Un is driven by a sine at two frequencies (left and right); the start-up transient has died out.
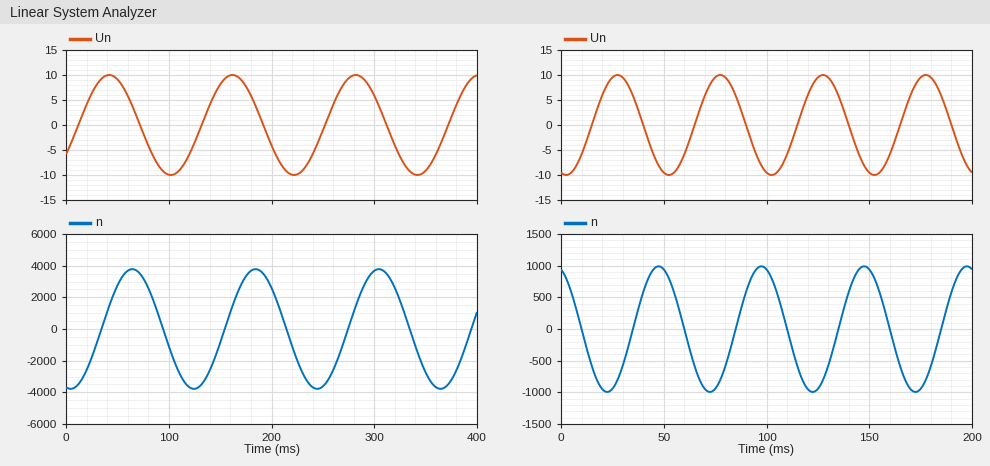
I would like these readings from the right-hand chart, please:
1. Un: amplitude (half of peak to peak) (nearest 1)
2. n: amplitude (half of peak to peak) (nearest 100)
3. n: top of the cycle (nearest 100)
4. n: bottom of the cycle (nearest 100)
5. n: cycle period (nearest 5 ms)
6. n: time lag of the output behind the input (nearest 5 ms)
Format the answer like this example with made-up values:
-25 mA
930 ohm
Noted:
10
1000
1000
-1000
50 ms
20 ms
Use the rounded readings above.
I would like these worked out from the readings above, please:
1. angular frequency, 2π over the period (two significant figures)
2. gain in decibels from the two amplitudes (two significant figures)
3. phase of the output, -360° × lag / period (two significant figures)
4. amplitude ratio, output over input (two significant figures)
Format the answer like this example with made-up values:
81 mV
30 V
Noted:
0.13 rad/ms
40 dB
-140°
100
